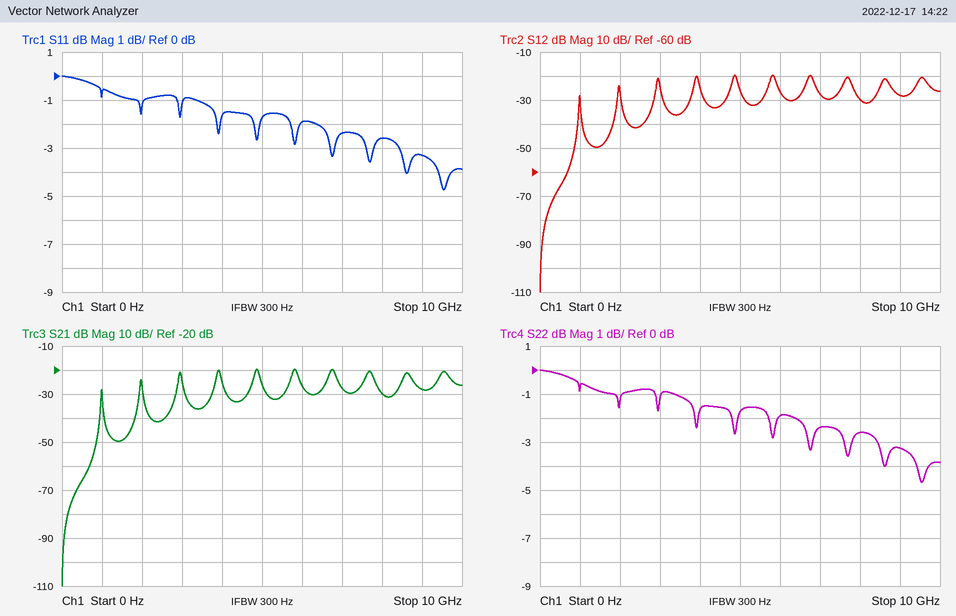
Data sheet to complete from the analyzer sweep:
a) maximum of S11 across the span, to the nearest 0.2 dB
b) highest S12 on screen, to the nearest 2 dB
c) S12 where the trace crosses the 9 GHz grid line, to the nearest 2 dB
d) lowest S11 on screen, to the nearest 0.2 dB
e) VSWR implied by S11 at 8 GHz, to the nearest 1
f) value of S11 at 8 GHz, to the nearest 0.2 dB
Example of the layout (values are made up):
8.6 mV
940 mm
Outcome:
0.0 dB
-20 dB
-28 dB
-4.8 dB
7
-2.6 dB
